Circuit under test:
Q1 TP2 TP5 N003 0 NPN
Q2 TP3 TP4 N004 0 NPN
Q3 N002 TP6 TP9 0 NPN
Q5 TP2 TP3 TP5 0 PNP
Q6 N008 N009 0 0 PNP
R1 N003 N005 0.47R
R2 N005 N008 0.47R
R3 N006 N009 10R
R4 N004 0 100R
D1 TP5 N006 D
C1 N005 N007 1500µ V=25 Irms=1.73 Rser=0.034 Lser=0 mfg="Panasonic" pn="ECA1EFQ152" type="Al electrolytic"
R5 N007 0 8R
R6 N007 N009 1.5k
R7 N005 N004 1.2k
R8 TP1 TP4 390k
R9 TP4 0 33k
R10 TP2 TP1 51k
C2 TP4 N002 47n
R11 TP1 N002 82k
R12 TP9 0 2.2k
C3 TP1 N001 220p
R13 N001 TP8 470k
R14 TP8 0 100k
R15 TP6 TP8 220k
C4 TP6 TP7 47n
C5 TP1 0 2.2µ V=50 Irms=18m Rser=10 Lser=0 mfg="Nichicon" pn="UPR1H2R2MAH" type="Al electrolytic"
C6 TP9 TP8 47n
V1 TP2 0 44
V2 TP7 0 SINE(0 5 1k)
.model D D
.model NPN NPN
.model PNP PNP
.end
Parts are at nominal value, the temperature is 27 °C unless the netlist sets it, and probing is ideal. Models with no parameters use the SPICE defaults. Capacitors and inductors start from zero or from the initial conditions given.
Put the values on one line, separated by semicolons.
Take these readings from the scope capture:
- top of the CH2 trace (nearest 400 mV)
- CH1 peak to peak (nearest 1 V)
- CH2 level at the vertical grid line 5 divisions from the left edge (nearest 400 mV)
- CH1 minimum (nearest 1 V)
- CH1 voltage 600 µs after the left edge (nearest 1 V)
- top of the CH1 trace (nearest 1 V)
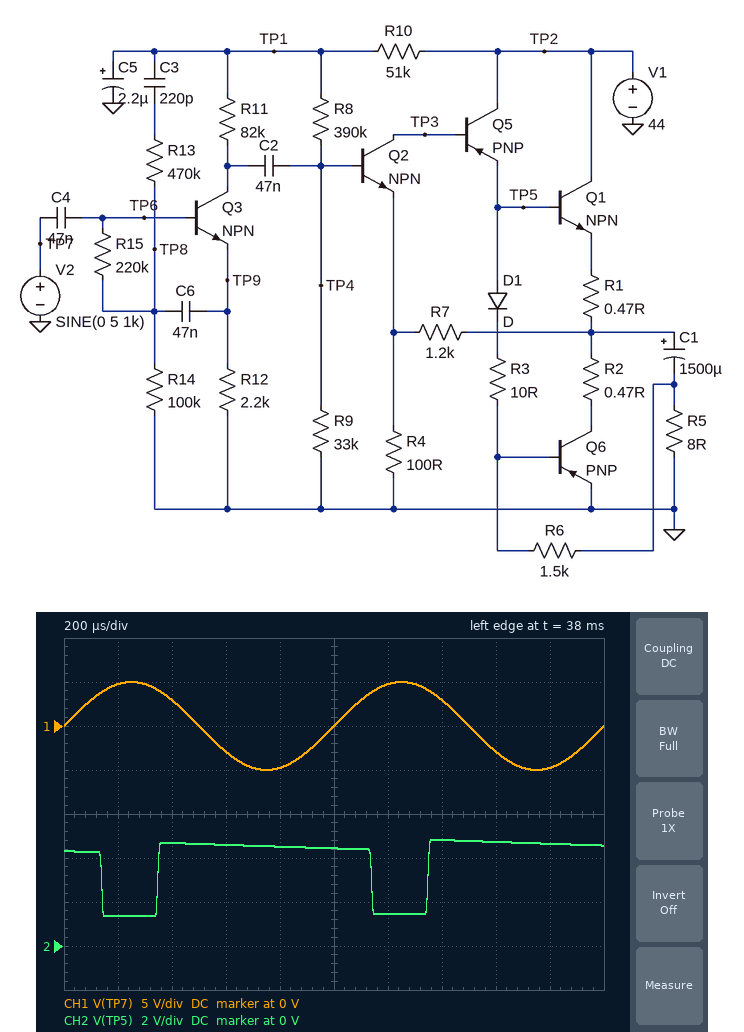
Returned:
4.8 V; 10 V; 4.4 V; -5 V; -3 V; 5 V
